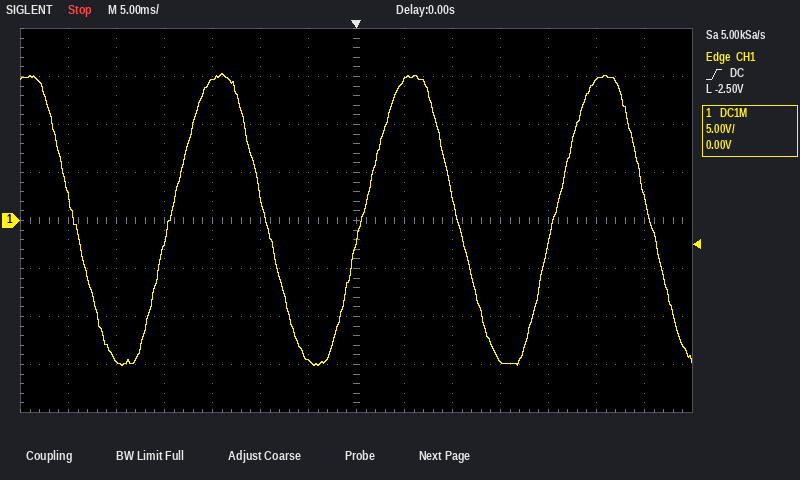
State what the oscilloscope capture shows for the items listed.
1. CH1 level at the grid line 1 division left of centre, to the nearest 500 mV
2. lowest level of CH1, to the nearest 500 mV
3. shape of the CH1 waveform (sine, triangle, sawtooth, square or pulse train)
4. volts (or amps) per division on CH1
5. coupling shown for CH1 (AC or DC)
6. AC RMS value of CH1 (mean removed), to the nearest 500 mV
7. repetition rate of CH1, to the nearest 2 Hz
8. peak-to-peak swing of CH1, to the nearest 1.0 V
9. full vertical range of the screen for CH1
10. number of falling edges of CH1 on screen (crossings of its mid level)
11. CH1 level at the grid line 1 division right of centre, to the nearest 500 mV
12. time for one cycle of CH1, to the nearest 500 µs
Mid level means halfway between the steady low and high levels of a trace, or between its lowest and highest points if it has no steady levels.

-14.5 V
-15.0 V
sine
5 V
DC
10.5 V
50 Hz
30.0 V
40 V
4
14.5 V
20.0 ms
